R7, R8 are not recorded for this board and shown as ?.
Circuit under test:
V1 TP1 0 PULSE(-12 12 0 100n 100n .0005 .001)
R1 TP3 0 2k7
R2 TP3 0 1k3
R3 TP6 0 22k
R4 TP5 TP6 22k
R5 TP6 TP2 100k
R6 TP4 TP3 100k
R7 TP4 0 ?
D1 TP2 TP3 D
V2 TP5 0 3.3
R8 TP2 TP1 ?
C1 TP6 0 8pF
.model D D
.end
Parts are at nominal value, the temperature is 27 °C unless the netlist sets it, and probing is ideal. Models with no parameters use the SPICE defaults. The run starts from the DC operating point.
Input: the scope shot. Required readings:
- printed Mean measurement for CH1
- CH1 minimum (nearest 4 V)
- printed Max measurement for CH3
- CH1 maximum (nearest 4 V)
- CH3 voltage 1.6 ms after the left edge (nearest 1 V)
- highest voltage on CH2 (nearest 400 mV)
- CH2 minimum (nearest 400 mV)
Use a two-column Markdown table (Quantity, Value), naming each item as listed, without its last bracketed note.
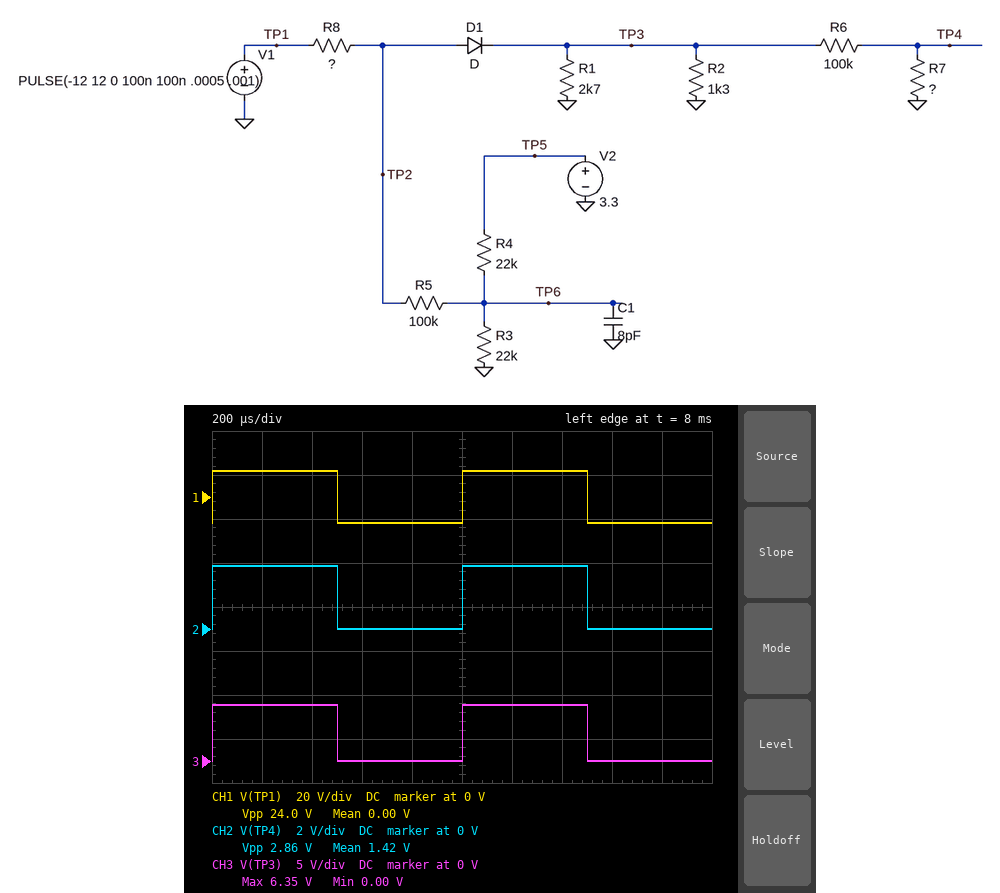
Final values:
| Quantity | Value |
|---|---|
| printed Mean measurement for CH1 | 0.00 V |
| CH1 minimum | -12 V |
| printed Max measurement for CH3 | 6.35 V |
| CH1 maximum | 12 V |
| CH3 voltage 1.6 ms after the left edge | 0 V |
| highest voltage on CH2 | 2.8 V |
| CH2 minimum | 0 V |
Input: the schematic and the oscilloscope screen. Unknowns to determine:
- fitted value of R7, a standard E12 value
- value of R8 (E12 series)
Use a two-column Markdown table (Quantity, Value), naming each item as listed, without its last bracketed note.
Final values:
| Quantity | Value |
|---|---|
| fitted value of R7, a standard E12 value | 82 kΩ |
| value of R8 | 680 Ω |
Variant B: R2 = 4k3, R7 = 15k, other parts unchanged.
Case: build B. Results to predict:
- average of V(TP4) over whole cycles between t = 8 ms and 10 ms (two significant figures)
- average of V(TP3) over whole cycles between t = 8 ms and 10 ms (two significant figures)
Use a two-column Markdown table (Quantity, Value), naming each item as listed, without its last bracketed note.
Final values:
| Quantity | Value |
|---|---|
| average of V(TP4) over whole cycles between t = 8 ms and 10 ms | 520 mV |
| average of V(TP3) over whole cycles between t = 8 ms and 10 ms | 4.0 V |
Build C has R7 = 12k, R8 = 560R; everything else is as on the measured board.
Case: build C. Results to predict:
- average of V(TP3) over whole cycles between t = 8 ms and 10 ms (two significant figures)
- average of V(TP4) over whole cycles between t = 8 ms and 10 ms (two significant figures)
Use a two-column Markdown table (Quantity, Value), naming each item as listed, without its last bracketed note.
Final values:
| Quantity | Value |
|---|---|
| average of V(TP3) over whole cycles between t = 8 ms and 10 ms | 3.4 V |
| average of V(TP4) over whole cycles between t = 8 ms and 10 ms | 370 mV |
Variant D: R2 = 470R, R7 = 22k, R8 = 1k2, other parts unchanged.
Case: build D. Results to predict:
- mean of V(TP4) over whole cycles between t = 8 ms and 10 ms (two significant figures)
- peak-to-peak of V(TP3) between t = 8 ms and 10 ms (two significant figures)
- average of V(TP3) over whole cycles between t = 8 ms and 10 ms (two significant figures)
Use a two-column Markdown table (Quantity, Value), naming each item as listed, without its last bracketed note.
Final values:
| Quantity | Value |
|---|---|
| mean of V(TP4) over whole cycles between t = 8 ms and 10 ms | 250 mV |
| peak-to-peak of V(TP3) between t = 8 ms and 10 ms | 2.8 V |
| average of V(TP3) over whole cycles between t = 8 ms and 10 ms | 1.4 V |
